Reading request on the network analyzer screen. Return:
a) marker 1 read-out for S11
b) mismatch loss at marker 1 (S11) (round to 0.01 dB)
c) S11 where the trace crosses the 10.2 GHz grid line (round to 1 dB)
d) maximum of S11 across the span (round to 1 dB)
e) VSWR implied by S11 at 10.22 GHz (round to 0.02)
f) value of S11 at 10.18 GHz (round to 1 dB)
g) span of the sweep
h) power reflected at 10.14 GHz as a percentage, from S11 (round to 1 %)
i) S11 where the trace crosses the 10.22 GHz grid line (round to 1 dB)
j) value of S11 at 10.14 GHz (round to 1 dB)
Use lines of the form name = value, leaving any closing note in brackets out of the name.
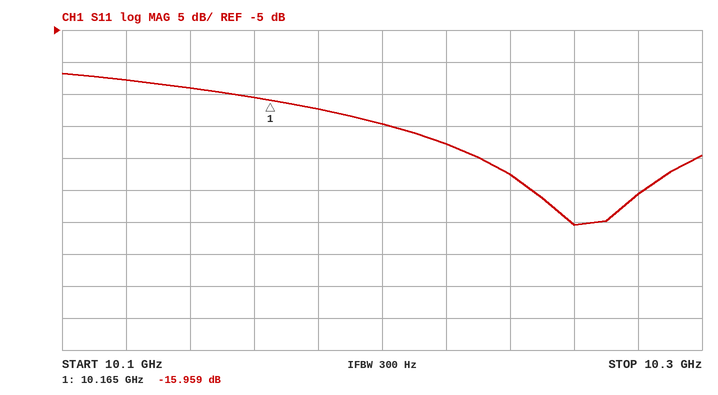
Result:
marker 1 read-out for S11 = -15.959 dB
mismatch loss at marker 1 (S11) = 0.11 dB
S11 where the trace crosses the 10.2 GHz grid line = -20 dB
maximum of S11 across the span = -12 dB
VSWR implied by S11 at 10.22 GHz = 1.16
value of S11 at 10.18 GHz = -17 dB
span of the sweep = 200 MHz
power reflected at 10.14 GHz as a percentage, from S11 = 4 %
S11 where the trace crosses the 10.22 GHz grid line = -23 dB
value of S11 at 10.14 GHz = -14 dB
